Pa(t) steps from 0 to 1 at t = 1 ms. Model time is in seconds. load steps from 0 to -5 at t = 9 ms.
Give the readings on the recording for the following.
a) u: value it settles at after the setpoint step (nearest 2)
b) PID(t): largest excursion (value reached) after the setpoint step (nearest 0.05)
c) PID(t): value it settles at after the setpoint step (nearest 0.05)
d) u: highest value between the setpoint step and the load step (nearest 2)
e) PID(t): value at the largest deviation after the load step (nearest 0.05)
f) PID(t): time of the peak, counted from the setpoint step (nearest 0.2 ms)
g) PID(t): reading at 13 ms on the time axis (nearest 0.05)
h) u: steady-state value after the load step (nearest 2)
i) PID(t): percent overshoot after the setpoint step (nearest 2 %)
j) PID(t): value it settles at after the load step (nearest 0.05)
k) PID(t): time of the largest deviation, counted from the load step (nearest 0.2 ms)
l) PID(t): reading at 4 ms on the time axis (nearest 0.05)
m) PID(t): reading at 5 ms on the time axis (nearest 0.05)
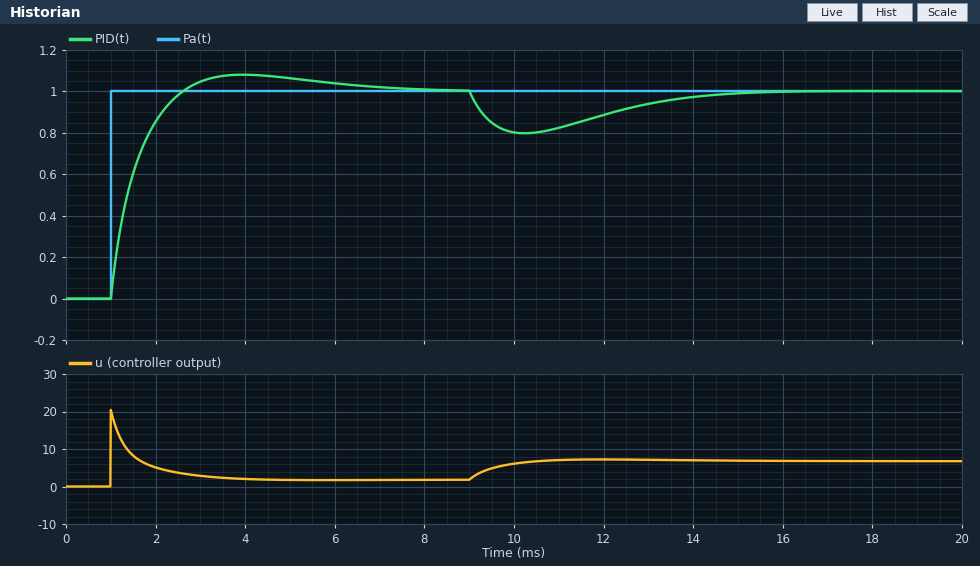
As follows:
2
1.10
1.00
20
0.80
3.0 ms
0.95
6
8 %
1.00
1.2 ms
1.10
1.05
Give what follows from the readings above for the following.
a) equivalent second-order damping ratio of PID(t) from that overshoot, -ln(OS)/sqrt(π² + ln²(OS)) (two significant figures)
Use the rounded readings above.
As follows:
0.63
